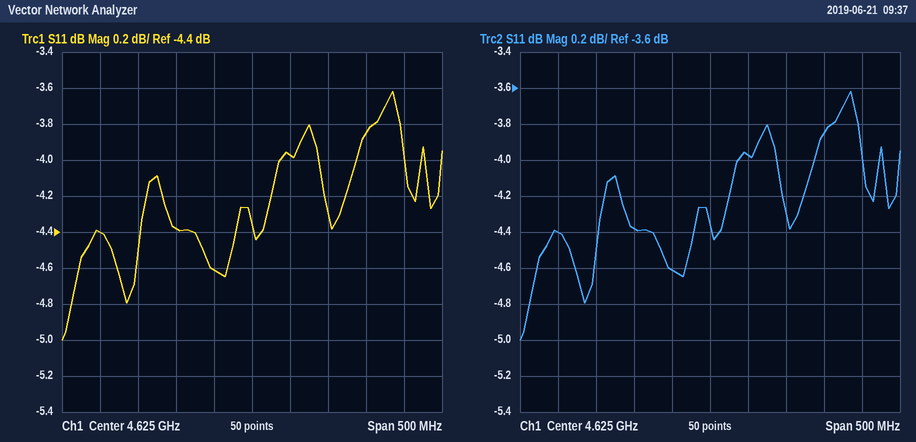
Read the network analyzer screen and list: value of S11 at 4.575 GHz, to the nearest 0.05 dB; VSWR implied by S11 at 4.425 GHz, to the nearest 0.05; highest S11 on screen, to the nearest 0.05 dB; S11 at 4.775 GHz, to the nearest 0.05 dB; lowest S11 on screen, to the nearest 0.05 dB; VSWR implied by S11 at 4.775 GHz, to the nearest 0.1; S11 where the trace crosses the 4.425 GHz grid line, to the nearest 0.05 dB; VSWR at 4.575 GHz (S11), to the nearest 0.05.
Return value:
-4.60 dB
4.05
-3.60 dB
-3.85 dB
-5.00 dB
4.6
-4.40 dB
3.85
